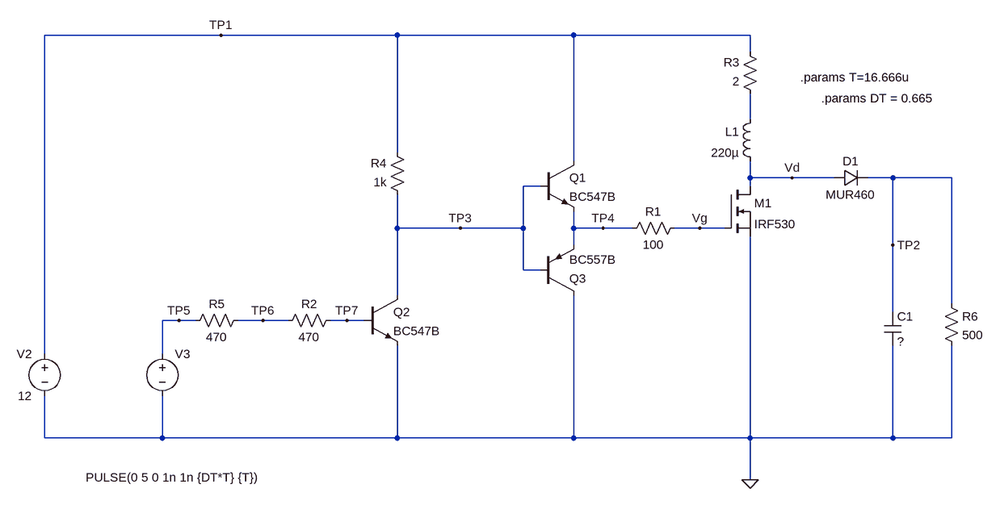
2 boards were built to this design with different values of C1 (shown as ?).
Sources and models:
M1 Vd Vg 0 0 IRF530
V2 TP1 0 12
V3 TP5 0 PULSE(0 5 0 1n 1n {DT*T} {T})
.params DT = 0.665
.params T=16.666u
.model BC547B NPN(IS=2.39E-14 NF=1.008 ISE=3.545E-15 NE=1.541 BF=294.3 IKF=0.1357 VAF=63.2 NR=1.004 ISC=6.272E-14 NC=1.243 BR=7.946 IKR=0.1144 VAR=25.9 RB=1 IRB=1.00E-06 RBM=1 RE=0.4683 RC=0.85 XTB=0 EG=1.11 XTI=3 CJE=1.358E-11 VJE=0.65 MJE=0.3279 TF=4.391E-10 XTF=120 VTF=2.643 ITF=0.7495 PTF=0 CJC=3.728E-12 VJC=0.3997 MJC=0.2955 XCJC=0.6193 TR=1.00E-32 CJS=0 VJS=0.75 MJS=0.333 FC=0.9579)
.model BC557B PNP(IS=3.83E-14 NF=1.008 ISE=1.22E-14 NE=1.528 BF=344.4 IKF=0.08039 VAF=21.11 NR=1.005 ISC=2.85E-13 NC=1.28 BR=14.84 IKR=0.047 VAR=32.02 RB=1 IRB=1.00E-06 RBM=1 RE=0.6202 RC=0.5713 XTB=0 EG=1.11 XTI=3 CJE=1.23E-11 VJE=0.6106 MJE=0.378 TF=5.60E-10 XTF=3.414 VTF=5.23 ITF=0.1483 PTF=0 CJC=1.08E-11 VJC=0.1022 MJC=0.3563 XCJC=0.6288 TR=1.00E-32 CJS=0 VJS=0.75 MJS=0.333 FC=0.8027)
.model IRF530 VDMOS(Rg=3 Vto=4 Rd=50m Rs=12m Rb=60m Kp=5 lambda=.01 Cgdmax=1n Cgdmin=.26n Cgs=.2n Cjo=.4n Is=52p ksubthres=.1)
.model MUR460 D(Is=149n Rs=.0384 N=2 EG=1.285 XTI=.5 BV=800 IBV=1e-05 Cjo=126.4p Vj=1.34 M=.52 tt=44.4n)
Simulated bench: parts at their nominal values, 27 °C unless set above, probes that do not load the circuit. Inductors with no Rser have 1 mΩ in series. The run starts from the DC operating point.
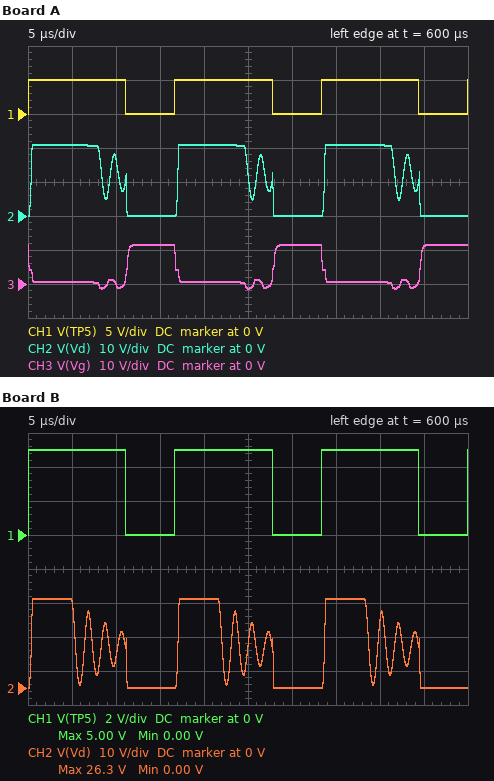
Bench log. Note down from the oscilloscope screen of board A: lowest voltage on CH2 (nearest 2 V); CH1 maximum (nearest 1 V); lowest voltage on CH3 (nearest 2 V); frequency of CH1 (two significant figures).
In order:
0 V
5 V
-2 V
60 kHz
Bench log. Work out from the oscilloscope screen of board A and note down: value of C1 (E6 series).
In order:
33 µF
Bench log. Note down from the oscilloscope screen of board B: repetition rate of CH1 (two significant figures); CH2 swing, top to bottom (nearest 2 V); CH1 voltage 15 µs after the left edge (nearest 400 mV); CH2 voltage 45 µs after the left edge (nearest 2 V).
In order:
60 kHz
26 V
0 V
0 V
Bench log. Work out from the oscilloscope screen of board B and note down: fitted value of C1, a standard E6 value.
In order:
15 µF
